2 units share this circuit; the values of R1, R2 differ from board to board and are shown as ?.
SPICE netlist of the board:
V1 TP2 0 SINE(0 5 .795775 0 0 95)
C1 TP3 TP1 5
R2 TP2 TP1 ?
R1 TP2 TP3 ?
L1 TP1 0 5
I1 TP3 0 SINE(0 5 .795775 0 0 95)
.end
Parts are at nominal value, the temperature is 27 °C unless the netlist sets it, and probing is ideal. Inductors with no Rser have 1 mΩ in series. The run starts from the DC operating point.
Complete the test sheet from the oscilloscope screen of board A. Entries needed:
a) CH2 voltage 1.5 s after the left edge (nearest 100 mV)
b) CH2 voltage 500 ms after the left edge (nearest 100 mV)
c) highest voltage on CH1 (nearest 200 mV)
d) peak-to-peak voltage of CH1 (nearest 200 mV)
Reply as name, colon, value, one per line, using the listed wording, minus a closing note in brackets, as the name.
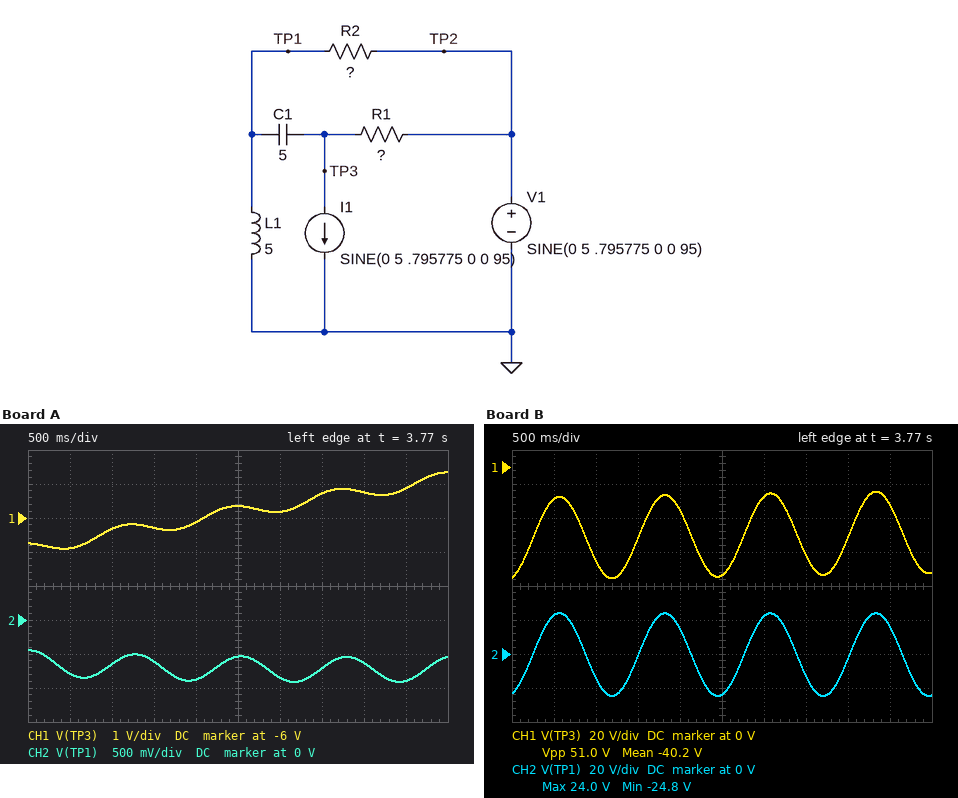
CH2 voltage 1.5 s after the left edge: -600 mV
CH2 voltage 500 ms after the left edge: -800 mV
highest voltage on CH1: -4.6 V
peak-to-peak voltage of CH1: 2.2 V
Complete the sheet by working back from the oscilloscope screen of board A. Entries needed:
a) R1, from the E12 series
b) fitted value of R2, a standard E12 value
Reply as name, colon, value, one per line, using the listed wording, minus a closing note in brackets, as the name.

R1, from the E12 series: 2.7 Ω
fitted value of R2, a standard E12 value: 1.5 Ω
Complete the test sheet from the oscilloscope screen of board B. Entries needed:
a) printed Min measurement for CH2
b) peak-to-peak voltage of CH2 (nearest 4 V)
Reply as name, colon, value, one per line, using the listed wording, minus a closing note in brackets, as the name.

printed Min measurement for CH2: -24.8 V
peak-to-peak voltage of CH2: 48 V
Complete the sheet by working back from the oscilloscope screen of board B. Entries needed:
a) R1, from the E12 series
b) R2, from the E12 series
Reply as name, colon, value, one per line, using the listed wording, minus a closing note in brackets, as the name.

R1, from the E12 series: 10 Ω
R2, from the E12 series: 15 Ω
